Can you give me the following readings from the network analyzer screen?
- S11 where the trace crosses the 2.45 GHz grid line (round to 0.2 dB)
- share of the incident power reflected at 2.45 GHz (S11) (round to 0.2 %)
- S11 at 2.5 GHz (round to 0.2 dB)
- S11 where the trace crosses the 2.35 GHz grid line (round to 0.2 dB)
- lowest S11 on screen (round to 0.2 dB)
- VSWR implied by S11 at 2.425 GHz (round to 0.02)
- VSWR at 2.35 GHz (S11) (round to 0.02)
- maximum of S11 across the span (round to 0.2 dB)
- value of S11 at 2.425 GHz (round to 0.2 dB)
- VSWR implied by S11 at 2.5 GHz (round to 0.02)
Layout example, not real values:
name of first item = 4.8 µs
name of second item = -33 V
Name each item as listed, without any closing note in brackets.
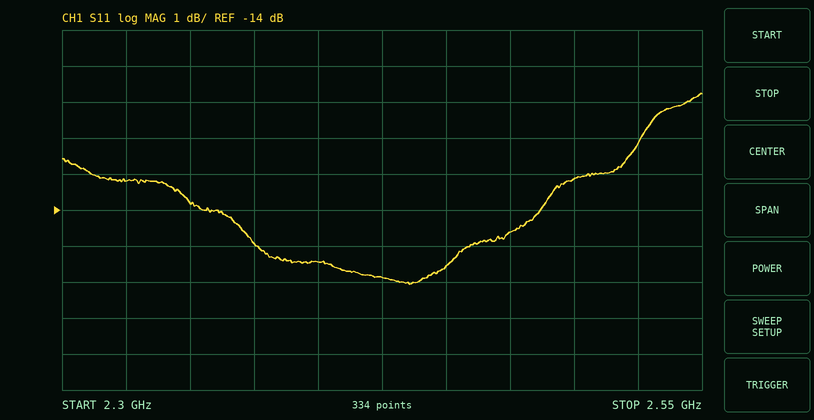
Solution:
S11 where the trace crosses the 2.45 GHz grid line = -15.6 dB
share of the incident power reflected at 2.45 GHz (S11) = 2.8 %
S11 at 2.5 GHz = -13.2 dB
S11 where the trace crosses the 2.35 GHz grid line = -13.8 dB
lowest S11 on screen = -16.0 dB
VSWR implied by S11 at 2.425 GHz = 1.38
VSWR at 2.35 GHz (S11) = 1.52
maximum of S11 across the span = -10.8 dB
value of S11 at 2.425 GHz = -15.8 dB
VSWR implied by S11 at 2.5 GHz = 1.56
